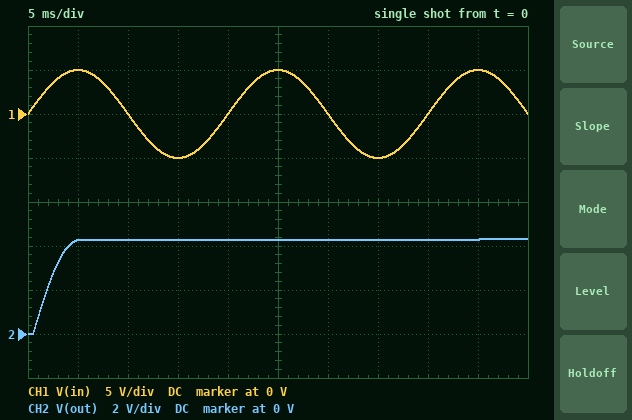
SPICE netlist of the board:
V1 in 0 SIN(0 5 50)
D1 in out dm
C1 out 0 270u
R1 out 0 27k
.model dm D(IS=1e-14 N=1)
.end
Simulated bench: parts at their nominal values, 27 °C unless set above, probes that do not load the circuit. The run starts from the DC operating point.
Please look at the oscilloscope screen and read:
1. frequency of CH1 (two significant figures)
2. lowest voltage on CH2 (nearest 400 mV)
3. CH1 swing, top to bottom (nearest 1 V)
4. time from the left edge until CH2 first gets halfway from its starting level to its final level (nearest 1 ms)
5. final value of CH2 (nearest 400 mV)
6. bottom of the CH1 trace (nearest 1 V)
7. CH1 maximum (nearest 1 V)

50 Hz
0 V
10 V
2 ms
4.4 V
-5 V
5 V
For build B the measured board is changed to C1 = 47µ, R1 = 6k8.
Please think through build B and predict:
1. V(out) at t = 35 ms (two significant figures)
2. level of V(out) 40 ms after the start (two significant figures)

4.2 V
4.1 V
